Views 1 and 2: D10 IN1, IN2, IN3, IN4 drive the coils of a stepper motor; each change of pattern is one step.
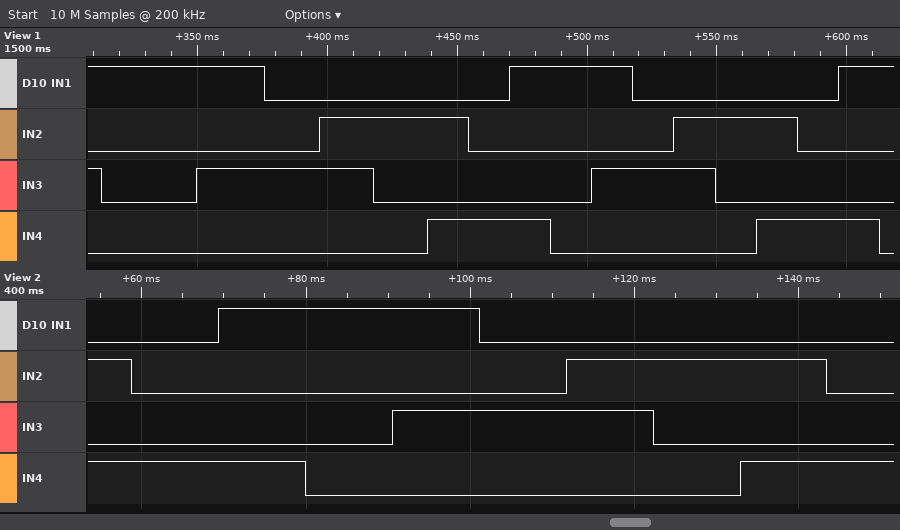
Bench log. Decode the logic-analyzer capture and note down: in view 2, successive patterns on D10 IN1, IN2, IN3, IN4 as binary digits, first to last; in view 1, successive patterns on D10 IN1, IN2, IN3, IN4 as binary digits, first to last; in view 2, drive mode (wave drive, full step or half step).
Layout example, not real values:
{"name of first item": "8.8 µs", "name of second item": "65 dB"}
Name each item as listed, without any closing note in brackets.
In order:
{"in view 2, successive patterns on D10 IN1, IN2, IN3, IN4 as binary digits, first to last": "0101 0001 1001 1000 1010 0010 0110 0100 0101 0001", "in view 1, successive patterns on D10 IN1, IN2, IN3, IN4 as binary digits, first to last": "1010 1000 1010 0010 0110 0100 0101 0001 1001 1000 1010 0010 0110 0100 0101 0001 1001 1000", "in view 2, drive mode": "half step"}
